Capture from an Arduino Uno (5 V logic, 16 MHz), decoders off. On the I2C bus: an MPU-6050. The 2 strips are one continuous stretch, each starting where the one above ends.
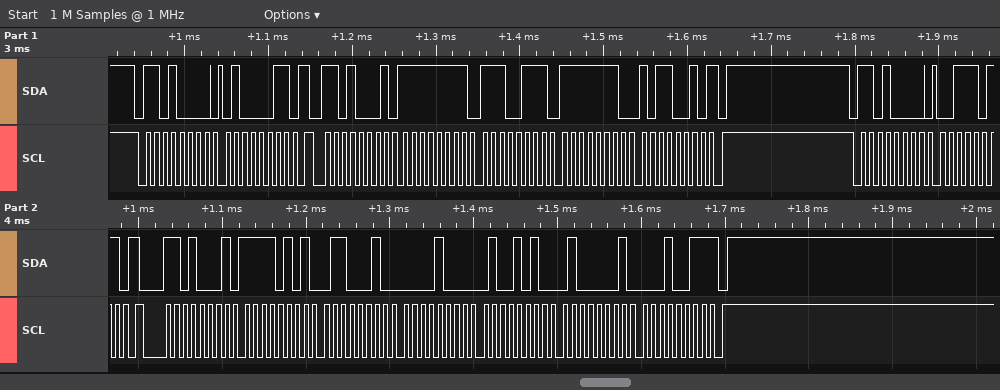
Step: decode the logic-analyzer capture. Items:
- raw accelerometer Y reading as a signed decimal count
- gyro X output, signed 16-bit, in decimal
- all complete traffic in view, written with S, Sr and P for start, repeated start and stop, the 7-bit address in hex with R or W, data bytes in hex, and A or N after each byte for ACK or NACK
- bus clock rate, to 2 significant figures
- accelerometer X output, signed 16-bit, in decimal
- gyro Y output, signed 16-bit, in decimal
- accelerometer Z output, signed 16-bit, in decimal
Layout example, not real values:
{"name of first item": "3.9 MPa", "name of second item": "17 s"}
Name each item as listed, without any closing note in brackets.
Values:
{"raw accelerometer Y reading as a signed decimal count": "2122", "gyro X output, signed 16-bit, in decimal": "-25", "all complete traffic in view, written with S, Sr and P for start, repeated start and stop, the 7-bit address in hex with R or W, data bytes in hex, and A or N after each byte for ACK or NACK": "S 68W A 43 A Sr 68R A FF A E7 A FE A B2 N P S 68W A 3B A Sr 68R A F5 A 62 A 08 A 4A A 41 A 13 N P", "bus clock rate, to 2 significant figures": "100 kHz", "accelerometer X output, signed 16-bit, in decimal": "-2718", "gyro Y output, signed 16-bit, in decimal": "-334", "accelerometer Z output, signed 16-bit, in decimal": "16659"}
